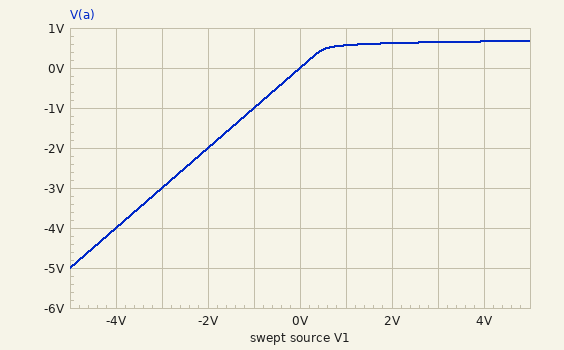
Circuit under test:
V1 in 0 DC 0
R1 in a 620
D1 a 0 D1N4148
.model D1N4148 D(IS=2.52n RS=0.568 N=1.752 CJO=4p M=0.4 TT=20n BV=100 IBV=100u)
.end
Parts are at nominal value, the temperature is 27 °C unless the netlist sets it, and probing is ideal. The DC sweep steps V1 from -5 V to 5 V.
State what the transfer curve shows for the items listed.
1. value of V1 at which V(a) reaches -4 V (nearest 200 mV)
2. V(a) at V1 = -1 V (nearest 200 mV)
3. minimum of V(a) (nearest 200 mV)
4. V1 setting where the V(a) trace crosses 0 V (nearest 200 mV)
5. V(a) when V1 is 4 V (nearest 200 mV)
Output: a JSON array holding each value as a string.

["-4.0 V", "-1.0 V", "-5.0 V", "0 V", "600 mV"]
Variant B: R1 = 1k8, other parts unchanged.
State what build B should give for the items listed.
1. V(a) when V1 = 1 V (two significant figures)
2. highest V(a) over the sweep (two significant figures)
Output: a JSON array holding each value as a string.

["520 mV", "630 mV"]
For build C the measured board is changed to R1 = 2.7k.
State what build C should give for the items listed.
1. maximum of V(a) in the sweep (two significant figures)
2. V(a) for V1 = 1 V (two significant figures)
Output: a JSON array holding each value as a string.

["610 mV", "510 mV"]
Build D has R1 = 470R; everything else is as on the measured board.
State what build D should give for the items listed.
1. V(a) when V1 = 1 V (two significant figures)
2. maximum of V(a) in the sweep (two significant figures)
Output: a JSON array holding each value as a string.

["580 mV", "690 mV"]
